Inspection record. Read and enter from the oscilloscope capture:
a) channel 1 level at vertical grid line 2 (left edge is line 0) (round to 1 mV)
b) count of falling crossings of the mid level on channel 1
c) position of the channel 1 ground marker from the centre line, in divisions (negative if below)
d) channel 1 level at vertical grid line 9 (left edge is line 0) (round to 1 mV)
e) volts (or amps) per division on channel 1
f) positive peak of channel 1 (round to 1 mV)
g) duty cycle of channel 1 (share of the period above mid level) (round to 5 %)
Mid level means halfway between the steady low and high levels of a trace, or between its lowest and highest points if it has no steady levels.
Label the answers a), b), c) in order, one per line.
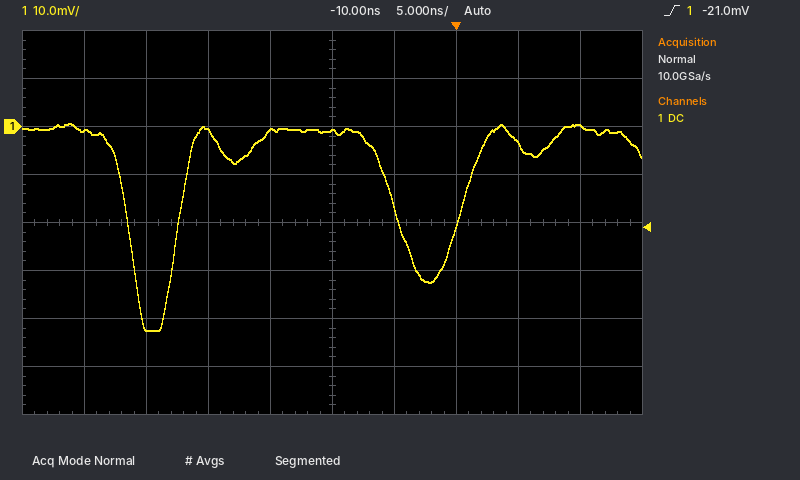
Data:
a) -42 mV
b) 2
c) +2.0 div
d) 0 mV
e) 10 mV
f) 1 mV
g) 80 %
